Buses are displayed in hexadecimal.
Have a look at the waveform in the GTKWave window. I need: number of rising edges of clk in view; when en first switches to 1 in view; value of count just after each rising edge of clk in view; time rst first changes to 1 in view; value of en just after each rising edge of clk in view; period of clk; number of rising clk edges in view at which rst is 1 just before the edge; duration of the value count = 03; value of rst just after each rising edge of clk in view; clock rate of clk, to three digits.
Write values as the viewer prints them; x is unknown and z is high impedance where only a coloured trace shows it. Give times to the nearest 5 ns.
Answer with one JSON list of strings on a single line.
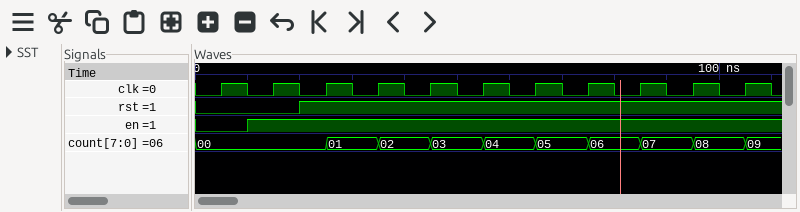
["11", "10 ns", "00, 00, 01, 02, 03, 04, 05, 06, 07, 08, 09", "20 ns", "0 1 1 1 1 1 1 1 1 1 1", "10 ns", "9", "10 ns", "0 0 1 1 1 1 1 1 1 1 1", "100 MHz"]
